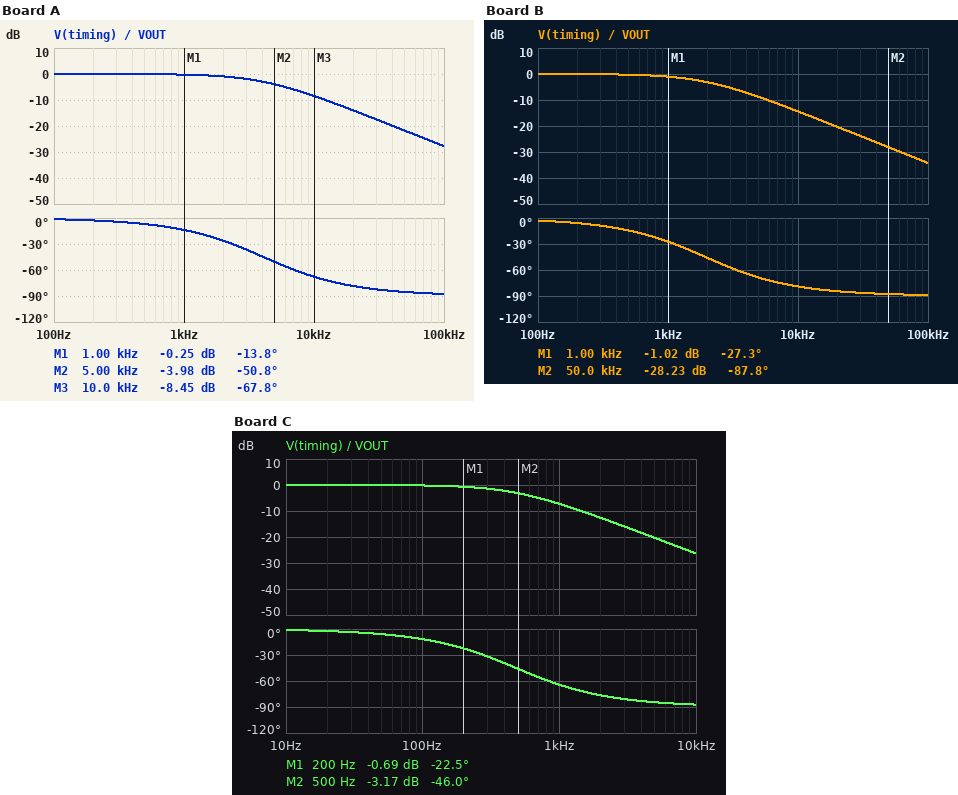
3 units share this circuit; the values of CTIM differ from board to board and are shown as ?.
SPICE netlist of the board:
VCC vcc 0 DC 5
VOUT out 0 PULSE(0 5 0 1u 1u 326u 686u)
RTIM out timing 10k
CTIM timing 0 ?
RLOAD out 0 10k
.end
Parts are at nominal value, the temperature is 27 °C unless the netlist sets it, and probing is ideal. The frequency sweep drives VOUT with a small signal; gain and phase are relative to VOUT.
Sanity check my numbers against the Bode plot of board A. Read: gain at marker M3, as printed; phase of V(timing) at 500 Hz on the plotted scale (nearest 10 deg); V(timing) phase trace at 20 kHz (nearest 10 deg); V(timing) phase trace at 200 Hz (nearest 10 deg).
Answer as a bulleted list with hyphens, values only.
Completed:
- -8.45 dB
- -10 deg
- -80 deg
- 0 deg
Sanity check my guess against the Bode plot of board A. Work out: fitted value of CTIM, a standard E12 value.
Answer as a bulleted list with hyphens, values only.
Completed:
- 3.9 nF
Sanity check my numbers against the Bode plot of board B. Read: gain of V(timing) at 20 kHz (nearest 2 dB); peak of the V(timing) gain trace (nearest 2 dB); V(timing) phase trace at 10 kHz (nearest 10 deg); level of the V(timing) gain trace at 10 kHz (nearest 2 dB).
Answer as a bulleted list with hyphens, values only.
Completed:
- -20 dB
- 0 dB
- -80 deg
- -14 dB
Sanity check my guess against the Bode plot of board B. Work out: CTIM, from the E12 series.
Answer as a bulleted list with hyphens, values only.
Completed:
- 8.2 nF
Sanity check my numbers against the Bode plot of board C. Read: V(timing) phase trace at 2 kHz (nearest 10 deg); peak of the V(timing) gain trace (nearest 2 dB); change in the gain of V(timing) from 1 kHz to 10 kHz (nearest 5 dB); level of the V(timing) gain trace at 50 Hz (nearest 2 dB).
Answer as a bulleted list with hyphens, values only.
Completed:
- -80 deg
- 0 dB
- -20 dB
- 0 dB
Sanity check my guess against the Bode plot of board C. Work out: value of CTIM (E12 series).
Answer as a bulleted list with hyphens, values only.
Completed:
- 33 nF
